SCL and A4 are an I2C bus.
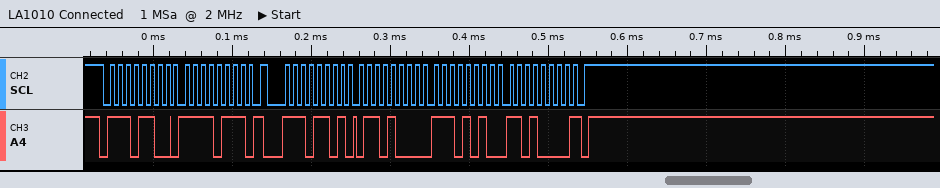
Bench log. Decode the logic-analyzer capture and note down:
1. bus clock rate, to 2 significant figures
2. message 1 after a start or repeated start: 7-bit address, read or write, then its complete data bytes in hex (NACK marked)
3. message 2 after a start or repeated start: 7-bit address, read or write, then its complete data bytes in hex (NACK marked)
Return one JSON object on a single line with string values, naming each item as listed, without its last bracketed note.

{"bus clock rate, to 2 significant figures": "100 kHz", "message 1 after a start or repeated start: 7-bit address, read or write, then its complete data bytes in hex": "0x76 write: F7", "message 2 after a start or repeated start: 7-bit address, read or write, then its complete data bytes in hex": "0x76 read: 68 EA D0 NACK"}
